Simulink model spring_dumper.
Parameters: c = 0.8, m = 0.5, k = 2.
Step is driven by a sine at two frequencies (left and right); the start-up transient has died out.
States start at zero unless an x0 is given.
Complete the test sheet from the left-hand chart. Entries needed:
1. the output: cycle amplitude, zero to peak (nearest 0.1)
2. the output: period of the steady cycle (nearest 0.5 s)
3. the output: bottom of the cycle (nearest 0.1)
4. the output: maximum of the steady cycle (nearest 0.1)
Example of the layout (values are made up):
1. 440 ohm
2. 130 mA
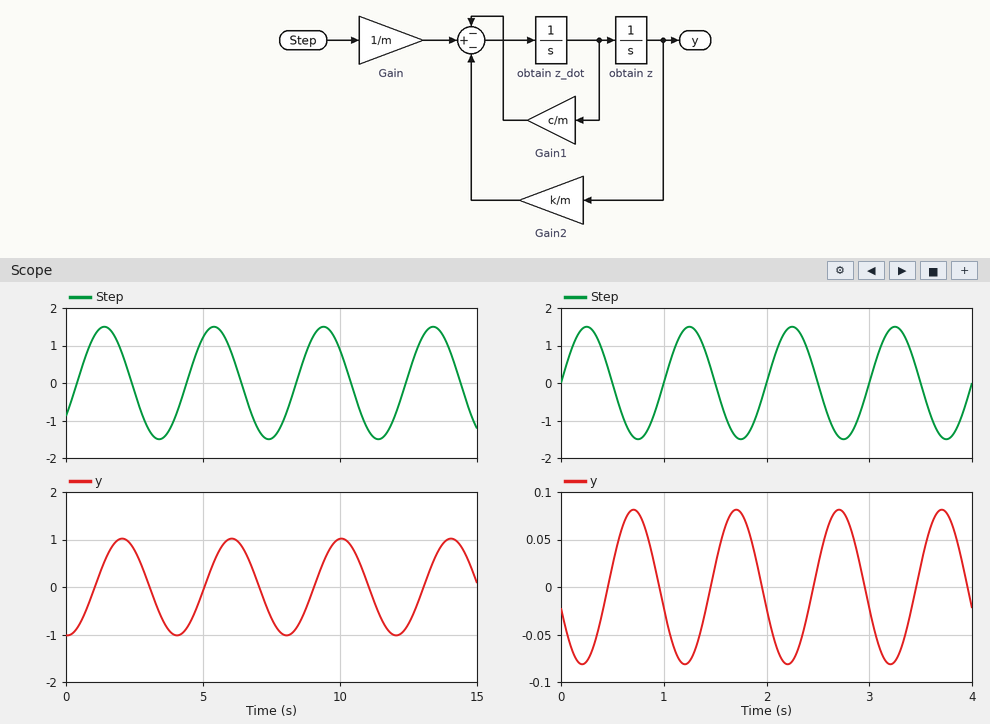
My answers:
1. 1.0
2. 4.0 s
3. -1.0
4. 1.0
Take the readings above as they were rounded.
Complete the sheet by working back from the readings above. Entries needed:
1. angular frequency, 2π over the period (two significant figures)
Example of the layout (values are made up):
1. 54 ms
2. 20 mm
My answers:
1. 1.6 rad/s
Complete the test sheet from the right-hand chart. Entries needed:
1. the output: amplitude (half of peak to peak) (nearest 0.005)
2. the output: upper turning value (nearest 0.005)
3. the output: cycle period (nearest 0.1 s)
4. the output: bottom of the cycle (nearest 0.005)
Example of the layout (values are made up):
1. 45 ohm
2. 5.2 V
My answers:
1. 0.080
2. 0.080
3. 1.0 s
4. -0.080
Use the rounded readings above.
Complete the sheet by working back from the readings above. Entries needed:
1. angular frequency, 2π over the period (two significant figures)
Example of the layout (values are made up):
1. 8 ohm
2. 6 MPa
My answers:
1. 6.3 rad/s
